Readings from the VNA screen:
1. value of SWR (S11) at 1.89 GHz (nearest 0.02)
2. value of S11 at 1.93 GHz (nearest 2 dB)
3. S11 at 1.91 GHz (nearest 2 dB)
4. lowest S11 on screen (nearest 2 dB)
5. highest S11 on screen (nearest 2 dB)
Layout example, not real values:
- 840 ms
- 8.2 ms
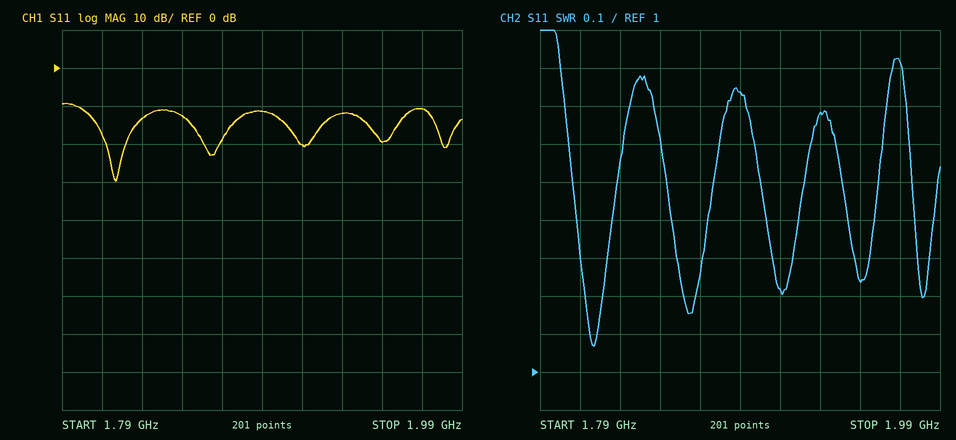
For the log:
- 1.74
- -12 dB
- -20 dB
- -30 dB
- -10 dB
